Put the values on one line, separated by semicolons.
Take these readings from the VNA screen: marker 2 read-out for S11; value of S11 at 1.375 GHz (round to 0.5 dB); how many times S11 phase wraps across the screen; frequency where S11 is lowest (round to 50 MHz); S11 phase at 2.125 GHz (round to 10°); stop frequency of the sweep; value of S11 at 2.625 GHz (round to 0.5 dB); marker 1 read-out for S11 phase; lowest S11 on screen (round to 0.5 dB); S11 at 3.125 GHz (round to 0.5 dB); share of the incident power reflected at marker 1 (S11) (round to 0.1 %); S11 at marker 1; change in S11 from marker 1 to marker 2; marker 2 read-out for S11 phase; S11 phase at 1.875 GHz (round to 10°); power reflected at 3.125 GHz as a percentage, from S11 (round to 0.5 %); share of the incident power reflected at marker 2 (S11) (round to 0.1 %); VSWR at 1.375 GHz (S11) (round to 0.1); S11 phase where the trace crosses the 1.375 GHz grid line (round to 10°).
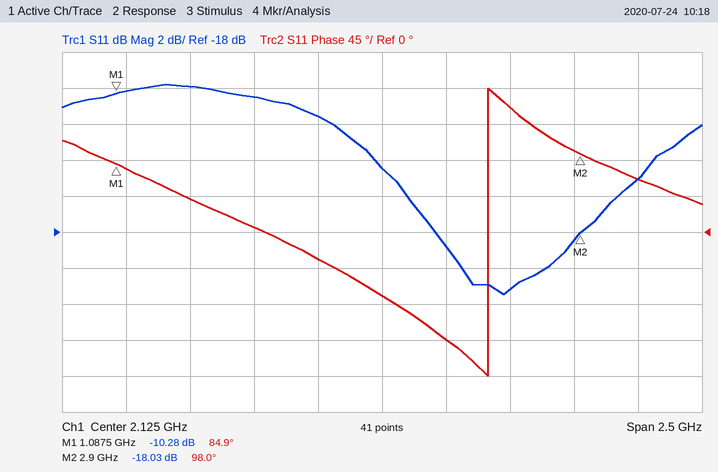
-18.03 dB; -10.0 dB; 1; 2.60 GHz; -80°; 3.375 GHz; -21.0 dB; 84.9°; -21.5 dB; -15.0 dB; 9.4 %; -10.28 dB; -7.75 dB; 98.0°; -30°; 3.0 %; 1.6 %; 1.9; 40°
